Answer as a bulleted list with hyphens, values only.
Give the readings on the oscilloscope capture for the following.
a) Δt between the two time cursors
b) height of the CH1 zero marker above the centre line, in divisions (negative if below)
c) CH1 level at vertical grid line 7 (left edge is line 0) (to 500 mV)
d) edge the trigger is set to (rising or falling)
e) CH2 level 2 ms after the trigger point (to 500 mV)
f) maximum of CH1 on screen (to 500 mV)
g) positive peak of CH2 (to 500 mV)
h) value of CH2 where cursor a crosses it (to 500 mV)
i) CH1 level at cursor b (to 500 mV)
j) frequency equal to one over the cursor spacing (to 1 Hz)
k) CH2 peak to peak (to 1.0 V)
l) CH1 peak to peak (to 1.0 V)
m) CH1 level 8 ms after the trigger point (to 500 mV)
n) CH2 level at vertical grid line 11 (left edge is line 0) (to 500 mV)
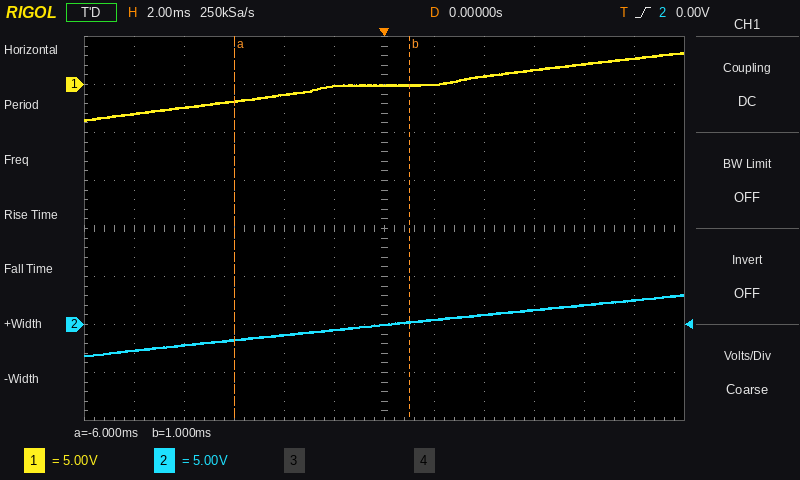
- 7.0 ms
- +3.0 div
- 0.0 V
- rising
- 500 mV
- 3.5 V
- 3.0 V
- -1.5 V
- 0.0 V
- 143 Hz
- 6.0 V
- 7.0 V
- 2.0 V
- 2.5 V
